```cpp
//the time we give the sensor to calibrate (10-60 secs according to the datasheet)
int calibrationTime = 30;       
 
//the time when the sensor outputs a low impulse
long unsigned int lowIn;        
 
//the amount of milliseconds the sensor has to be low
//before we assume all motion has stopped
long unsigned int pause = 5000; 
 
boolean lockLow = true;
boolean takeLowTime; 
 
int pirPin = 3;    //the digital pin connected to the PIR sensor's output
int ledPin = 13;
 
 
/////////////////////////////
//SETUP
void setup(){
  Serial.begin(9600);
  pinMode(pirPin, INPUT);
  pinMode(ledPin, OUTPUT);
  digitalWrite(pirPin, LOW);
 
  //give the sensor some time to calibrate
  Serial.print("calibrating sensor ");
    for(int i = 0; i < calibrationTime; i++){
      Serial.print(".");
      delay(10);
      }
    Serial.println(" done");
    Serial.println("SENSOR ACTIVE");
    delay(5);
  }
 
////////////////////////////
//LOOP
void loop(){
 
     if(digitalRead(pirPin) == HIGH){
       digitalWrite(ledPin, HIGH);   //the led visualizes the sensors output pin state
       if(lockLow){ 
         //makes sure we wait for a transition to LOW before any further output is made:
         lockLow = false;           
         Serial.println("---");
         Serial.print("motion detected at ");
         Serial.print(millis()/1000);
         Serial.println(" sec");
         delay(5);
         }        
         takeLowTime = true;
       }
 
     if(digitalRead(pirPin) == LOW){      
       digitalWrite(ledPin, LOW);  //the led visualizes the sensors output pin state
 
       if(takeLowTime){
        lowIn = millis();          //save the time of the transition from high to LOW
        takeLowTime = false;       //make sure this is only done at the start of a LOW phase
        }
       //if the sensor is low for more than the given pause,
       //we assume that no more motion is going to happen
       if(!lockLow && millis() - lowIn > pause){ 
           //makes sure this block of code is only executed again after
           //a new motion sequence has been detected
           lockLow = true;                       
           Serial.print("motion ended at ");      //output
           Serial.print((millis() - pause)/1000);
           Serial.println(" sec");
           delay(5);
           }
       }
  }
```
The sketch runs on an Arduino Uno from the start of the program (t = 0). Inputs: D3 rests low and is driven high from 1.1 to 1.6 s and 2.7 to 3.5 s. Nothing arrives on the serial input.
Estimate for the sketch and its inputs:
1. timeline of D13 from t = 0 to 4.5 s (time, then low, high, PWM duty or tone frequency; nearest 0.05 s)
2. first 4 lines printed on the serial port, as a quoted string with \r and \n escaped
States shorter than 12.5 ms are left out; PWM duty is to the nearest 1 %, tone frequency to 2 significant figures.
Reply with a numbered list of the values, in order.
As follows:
1. 0 s low; 1.1 s high; 1.6 s low; 2.7 s high; 3.5 s low
2. "calibrating sensor .............................. done\r\nSENSOR ACTIVE\r\n---\r\nmotion detected at 1 sec\r\n"
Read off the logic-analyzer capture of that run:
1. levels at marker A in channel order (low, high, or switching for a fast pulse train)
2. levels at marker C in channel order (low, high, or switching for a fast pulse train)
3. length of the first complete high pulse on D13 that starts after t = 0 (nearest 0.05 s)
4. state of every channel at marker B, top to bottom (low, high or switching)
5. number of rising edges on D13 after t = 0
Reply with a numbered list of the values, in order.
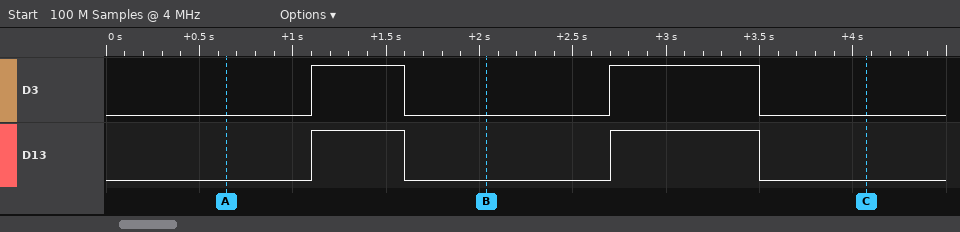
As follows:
1. D3 low, D13 low
2. D3 low, D13 low
3. 0.50 s
4. D3 low, D13 low
5. 2
